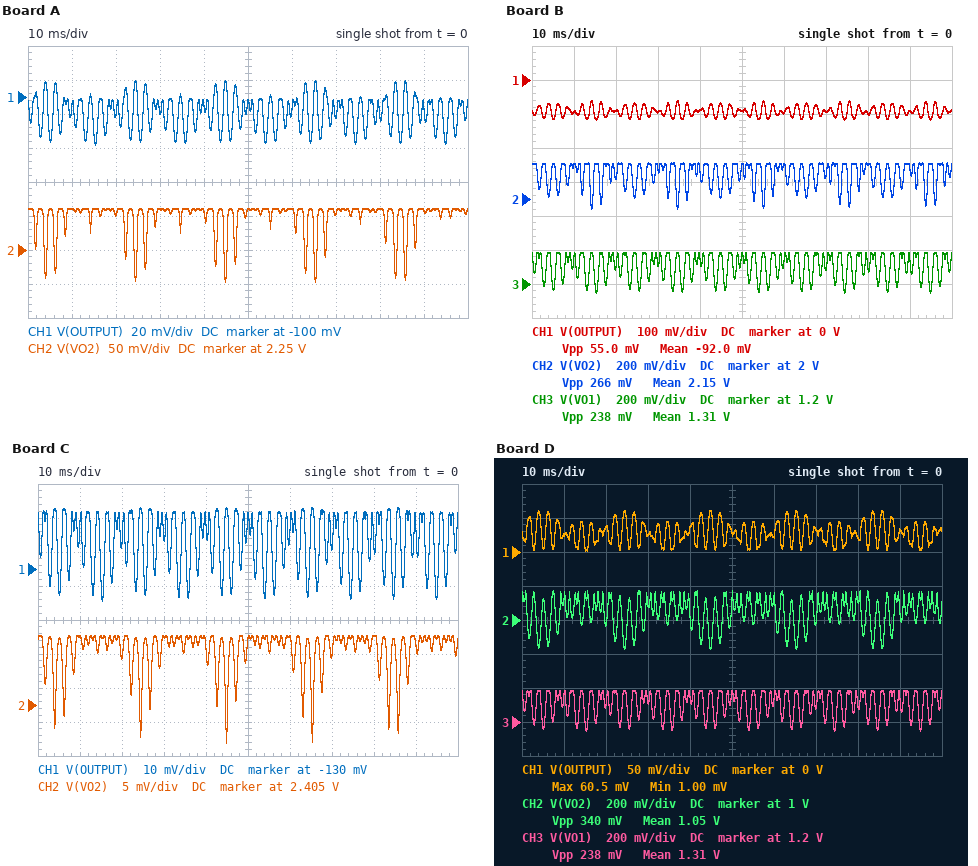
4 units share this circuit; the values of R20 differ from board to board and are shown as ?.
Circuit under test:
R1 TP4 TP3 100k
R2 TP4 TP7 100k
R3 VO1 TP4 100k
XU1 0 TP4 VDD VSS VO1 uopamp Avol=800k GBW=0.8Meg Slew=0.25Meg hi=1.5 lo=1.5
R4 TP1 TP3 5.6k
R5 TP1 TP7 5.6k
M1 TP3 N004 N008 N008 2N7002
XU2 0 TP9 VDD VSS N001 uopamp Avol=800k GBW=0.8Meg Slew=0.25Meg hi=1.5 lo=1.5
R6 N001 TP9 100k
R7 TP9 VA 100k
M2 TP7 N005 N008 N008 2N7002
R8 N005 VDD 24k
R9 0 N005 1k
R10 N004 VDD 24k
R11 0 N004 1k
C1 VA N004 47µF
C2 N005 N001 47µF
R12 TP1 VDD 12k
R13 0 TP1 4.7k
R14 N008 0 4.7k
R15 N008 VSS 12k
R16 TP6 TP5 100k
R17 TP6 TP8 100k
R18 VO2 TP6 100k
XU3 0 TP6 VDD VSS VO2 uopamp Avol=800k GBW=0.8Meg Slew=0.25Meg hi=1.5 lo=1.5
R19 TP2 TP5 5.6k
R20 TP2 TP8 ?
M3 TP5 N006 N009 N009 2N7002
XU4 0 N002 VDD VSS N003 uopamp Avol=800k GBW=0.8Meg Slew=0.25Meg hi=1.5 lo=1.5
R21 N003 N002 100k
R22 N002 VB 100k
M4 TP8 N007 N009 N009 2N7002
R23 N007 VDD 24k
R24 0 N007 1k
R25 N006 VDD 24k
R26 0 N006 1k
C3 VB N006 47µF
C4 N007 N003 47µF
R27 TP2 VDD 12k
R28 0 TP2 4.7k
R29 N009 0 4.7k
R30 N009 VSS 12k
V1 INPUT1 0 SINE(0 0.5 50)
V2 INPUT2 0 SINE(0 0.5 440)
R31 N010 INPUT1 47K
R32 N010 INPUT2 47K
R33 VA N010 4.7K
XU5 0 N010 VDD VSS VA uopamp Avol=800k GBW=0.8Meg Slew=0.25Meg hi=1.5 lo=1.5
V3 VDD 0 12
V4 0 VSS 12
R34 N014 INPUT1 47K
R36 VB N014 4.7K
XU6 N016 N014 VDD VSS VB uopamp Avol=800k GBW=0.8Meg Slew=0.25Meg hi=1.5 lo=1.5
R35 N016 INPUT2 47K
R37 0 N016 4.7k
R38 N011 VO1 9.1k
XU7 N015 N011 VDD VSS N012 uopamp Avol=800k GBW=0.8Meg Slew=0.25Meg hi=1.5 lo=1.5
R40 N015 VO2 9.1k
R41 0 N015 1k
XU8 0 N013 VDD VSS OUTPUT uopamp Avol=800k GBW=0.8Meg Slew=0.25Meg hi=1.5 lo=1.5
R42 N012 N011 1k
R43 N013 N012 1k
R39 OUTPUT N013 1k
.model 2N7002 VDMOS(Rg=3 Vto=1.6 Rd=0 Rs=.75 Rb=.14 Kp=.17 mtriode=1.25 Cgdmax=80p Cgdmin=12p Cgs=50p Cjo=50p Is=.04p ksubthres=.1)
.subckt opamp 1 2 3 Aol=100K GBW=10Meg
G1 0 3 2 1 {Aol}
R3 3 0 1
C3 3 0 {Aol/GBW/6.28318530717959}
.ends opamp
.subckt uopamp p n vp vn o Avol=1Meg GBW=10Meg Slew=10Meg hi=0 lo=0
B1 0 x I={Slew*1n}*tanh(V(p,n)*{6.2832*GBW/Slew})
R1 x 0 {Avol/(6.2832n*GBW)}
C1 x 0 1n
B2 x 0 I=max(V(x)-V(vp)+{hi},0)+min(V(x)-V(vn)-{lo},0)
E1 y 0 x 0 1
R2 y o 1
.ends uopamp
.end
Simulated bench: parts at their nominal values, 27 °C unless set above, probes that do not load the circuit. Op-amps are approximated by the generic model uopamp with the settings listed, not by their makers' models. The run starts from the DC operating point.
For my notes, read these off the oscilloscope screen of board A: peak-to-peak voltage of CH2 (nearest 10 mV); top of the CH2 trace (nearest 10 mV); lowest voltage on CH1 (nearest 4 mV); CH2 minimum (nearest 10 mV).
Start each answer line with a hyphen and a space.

- 110 mV
- 2.31 V
- -128 mV
- 2.20 V
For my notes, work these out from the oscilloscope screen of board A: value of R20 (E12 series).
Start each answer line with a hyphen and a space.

- 12 kΩ
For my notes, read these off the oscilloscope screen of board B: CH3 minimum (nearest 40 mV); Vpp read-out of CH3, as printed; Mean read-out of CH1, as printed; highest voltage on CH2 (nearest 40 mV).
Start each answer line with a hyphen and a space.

- 1.16 V
- 238 mV
- -92.0 mV
- 2.20 V
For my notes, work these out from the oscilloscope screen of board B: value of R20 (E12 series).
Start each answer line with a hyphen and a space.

- 10 kΩ
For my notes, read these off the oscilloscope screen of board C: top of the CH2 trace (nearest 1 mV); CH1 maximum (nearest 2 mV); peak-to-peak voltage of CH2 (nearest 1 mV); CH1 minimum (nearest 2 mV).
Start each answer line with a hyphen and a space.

- 2.415 V
- -112 mV
- 16 mV
- -140 mV
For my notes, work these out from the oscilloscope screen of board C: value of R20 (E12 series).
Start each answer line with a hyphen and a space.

- 15 kΩ
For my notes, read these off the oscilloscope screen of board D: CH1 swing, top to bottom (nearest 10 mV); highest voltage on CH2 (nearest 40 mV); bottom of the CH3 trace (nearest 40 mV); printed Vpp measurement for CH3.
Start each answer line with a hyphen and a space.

- 60 mV
- 1.16 V
- 1.16 V
- 238 mV
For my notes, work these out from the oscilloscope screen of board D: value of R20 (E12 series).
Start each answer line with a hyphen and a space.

- 4.7 kΩ
